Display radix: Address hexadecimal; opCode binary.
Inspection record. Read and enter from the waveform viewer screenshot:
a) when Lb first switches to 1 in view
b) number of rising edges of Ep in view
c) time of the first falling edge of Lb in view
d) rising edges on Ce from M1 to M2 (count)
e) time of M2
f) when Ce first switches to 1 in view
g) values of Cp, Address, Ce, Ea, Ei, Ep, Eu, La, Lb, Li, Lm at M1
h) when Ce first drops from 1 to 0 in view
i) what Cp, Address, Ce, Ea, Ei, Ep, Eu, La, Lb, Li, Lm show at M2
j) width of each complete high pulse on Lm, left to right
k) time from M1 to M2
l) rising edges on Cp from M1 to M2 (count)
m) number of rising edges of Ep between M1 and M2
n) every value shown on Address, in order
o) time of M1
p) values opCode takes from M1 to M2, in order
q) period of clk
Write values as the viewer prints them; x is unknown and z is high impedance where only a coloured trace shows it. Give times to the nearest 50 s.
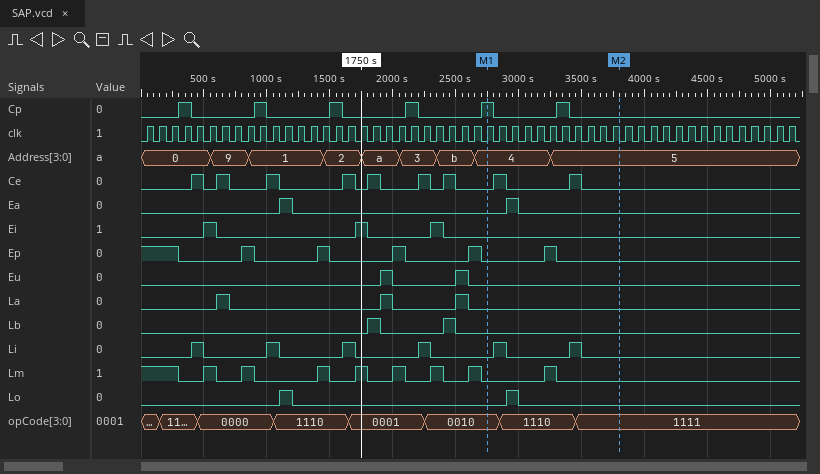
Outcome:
1800 s
5
1900 s
2
3800 s
400 s
Cp=1, Address=4, Ce=0, Ea=0, Ei=0, Ep=0, Eu=0, La=0, Lb=0, Li=0, Lm=0
500 s
Cp=0, Address=5, Ce=0, Ea=0, Ei=0, Ep=0, Eu=0, La=0, Lb=0, Li=0, Lm=0
100 s, 100 s, 100 s, 100 s, 100 s, 100 s, 100 s, 100 s
1050 s
1
1
0, 9, 1, 2, a, 3, b, 4, 5
2750 s
0010, 1110, 1111
100 s
